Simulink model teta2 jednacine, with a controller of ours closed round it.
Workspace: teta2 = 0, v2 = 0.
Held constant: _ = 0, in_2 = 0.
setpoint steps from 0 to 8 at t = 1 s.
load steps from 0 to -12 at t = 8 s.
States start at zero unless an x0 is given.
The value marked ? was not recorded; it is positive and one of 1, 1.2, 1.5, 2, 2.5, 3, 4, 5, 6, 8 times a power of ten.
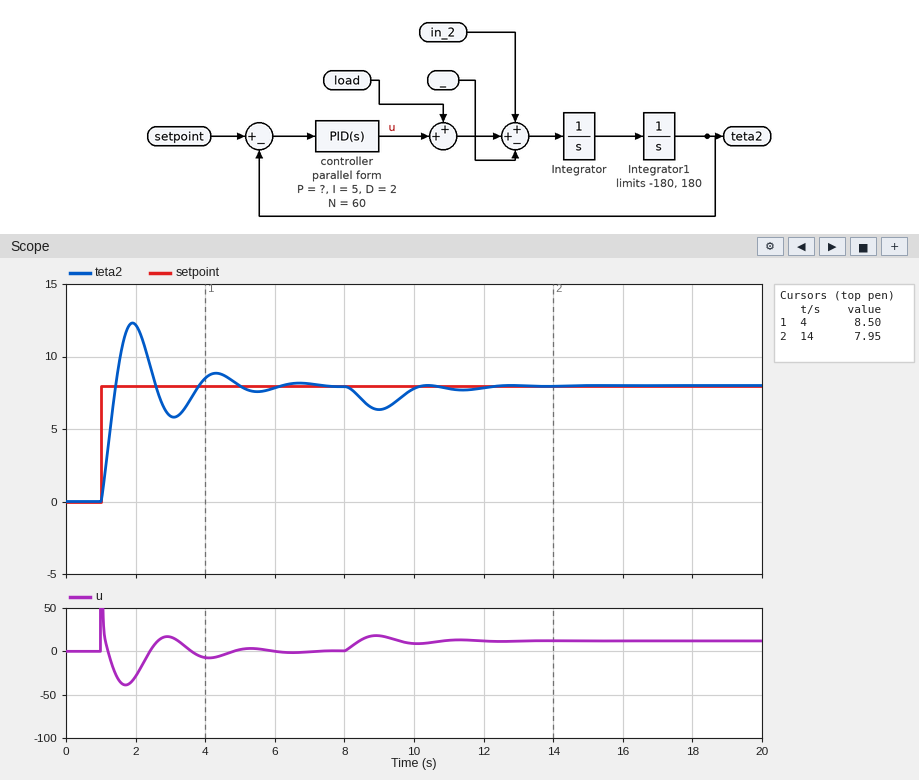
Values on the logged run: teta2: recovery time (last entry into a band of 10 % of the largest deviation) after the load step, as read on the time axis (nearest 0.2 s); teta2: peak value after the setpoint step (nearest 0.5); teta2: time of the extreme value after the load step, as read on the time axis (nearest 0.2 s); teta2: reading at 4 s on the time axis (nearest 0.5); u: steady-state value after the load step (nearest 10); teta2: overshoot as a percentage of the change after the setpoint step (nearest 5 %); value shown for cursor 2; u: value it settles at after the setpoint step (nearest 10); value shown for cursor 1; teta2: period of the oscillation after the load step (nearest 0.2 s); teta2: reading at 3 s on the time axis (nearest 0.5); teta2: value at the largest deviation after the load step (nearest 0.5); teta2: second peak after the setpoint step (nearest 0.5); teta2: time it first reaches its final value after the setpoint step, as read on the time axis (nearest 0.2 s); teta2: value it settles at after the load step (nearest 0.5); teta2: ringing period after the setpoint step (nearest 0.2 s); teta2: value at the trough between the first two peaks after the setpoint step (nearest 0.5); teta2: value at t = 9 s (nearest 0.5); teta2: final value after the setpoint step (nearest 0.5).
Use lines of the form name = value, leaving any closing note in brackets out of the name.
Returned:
teta2: recovery time (last entry into a band of 10 % of the largest deviation) after the load step, as read on the time axis = 12.0 s
teta2: peak value after the setpoint step = 12.5
teta2: time of the extreme value after the load step, as read on the time axis = 9.0 s
teta2: reading at 4 s on the time axis = 8.5
u: steady-state value after the load step = 10
teta2: overshoot as a percentage of the change after the setpoint step = 55 %
value shown for cursor 2 = 7.95
u: value it settles at after the setpoint step = 0
value shown for cursor 1 = 8.50
teta2: period of the oscillation after the load step = 2.4 s
teta2: reading at 3 s on the time axis = 6.0
teta2: value at the largest deviation after the load step = 6.5
teta2: second peak after the setpoint step = 9.0
teta2: time it first reaches its final value after the setpoint step, as read on the time axis = 1.4 s
teta2: value it settles at after the load step = 8.0
teta2: ringing period after the setpoint step = 2.4 s
teta2: value at the trough between the first two peaks after the setpoint step = 6.0
teta2: value at t = 9 s = 6.5
teta2: final value after the setpoint step = 8.0
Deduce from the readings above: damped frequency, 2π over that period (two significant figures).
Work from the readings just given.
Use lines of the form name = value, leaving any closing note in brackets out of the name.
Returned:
damped frequency, 2π over that period = 2.6 rad/s
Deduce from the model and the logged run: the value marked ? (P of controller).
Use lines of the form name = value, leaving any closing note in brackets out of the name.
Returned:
the value marked ? = 8
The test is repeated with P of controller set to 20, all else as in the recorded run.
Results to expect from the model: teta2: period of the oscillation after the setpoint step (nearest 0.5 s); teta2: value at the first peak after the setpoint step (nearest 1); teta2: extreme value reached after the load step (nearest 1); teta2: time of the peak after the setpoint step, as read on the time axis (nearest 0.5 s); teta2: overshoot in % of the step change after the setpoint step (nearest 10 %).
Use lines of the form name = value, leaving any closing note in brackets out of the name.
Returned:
teta2: period of the oscillation after the setpoint step = 1.5 s
teta2: value at the first peak after the setpoint step = 13
teta2: extreme value reached after the load step = 7
teta2: time of the peak after the setpoint step, as read on the time axis = 1.5 s
teta2: overshoot in % of the step change after the setpoint step = 60 %
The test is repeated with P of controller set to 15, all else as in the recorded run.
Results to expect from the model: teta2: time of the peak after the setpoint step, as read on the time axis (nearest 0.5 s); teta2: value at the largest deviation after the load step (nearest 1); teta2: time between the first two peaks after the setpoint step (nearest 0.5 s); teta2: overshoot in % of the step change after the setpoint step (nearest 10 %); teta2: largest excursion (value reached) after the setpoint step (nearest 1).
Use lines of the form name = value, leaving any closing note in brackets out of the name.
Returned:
teta2: time of the peak after the setpoint step, as read on the time axis = 1.5 s
teta2: value at the largest deviation after the load step = 7
teta2: time between the first two peaks after the setpoint step = 1.5 s
teta2: overshoot in % of the step change after the setpoint step = 60 %
teta2: largest excursion (value reached) after the setpoint step = 13
